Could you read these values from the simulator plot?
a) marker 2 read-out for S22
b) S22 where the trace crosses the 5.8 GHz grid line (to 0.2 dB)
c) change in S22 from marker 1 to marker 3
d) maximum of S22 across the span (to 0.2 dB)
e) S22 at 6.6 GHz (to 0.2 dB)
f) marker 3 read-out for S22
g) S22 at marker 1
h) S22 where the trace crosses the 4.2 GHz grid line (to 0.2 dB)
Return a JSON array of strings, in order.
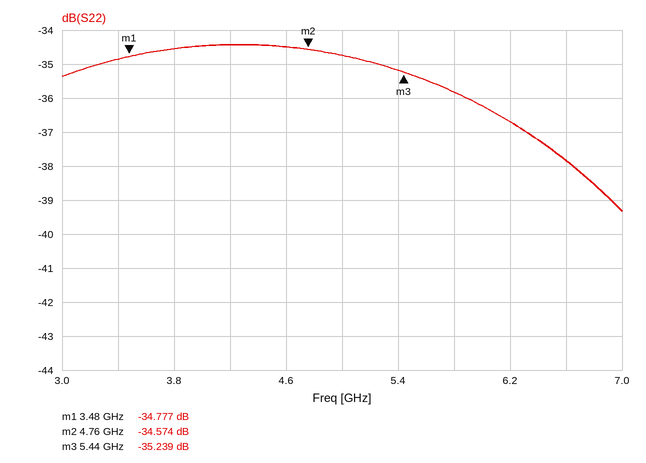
["-34.574 dB", "-35.8 dB", "-0.462 dB", "-34.4 dB", "-37.8 dB", "-35.239 dB", "-34.777 dB", "-34.4 dB"]
